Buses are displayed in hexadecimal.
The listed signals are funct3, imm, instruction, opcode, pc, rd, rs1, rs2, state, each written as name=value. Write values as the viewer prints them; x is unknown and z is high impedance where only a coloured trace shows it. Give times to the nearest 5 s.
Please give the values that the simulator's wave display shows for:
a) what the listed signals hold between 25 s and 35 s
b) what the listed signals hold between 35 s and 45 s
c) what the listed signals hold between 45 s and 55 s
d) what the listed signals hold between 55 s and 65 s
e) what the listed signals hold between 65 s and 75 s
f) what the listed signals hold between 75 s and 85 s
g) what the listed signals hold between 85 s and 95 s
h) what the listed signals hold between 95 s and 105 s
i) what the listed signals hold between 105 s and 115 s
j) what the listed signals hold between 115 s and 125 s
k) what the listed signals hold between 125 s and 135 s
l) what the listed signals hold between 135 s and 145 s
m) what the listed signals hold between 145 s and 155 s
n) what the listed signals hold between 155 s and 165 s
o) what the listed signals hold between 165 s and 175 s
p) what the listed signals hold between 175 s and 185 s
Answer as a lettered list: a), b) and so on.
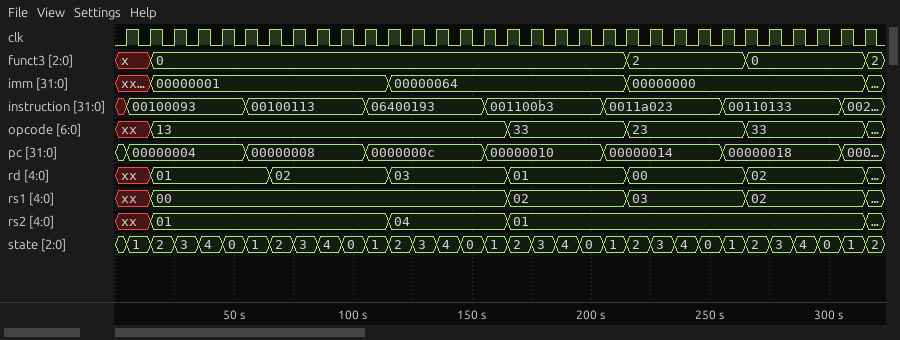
a) funct3=0, imm=00000001, instruction=00100093, opcode=13, pc=00000004, rd=01, rs1=00, rs2=01, state=3
b) funct3=0, imm=00000001, instruction=00100093, opcode=13, pc=00000004, rd=01, rs1=00, rs2=01, state=4
c) funct3=0, imm=00000001, instruction=00100093, opcode=13, pc=00000004, rd=01, rs1=00, rs2=01, state=0
d) funct3=0, imm=00000001, instruction=00100113, opcode=13, pc=00000008, rd=01, rs1=00, rs2=01, state=1
e) funct3=0, imm=00000001, instruction=00100113, opcode=13, pc=00000008, rd=02, rs1=00, rs2=01, state=2
f) funct3=0, imm=00000001, instruction=00100113, opcode=13, pc=00000008, rd=02, rs1=00, rs2=01, state=3
g) funct3=0, imm=00000001, instruction=00100113, opcode=13, pc=00000008, rd=02, rs1=00, rs2=01, state=4
h) funct3=0, imm=00000001, instruction=00100113, opcode=13, pc=00000008, rd=02, rs1=00, rs2=01, state=0
i) funct3=0, imm=00000001, instruction=06400193, opcode=13, pc=0000000c, rd=02, rs1=00, rs2=01, state=1
j) funct3=0, imm=00000064, instruction=06400193, opcode=13, pc=0000000c, rd=03, rs1=00, rs2=04, state=2
k) funct3=0, imm=00000064, instruction=06400193, opcode=13, pc=0000000c, rd=03, rs1=00, rs2=04, state=3
l) funct3=0, imm=00000064, instruction=06400193, opcode=13, pc=0000000c, rd=03, rs1=00, rs2=04, state=4
m) funct3=0, imm=00000064, instruction=06400193, opcode=13, pc=0000000c, rd=03, rs1=00, rs2=04, state=0
n) funct3=0, imm=00000064, instruction=001100b3, opcode=13, pc=00000010, rd=03, rs1=00, rs2=04, state=1
o) funct3=0, imm=00000064, instruction=001100b3, opcode=33, pc=00000010, rd=01, rs1=02, rs2=01, state=2
p) funct3=0, imm=00000064, instruction=001100b3, opcode=33, pc=00000010, rd=01, rs1=02, rs2=01, state=3
